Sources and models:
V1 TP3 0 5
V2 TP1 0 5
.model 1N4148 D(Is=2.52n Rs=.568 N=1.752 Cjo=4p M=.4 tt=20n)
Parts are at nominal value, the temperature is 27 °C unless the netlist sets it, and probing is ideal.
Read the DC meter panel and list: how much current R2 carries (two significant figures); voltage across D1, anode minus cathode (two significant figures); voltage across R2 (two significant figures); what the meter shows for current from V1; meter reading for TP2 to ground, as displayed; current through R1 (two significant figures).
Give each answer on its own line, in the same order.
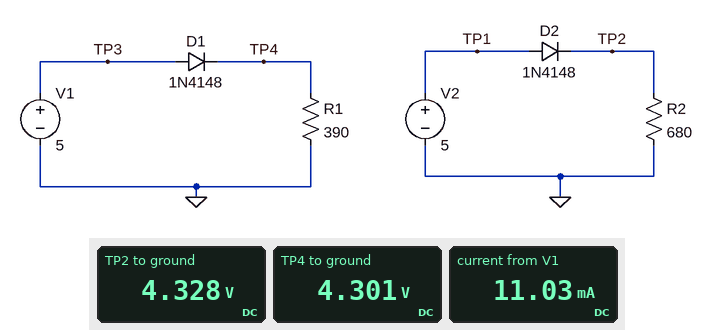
6.4 mA
700 mV
4.3 V
11.03 mA
4.328 V
11 mA
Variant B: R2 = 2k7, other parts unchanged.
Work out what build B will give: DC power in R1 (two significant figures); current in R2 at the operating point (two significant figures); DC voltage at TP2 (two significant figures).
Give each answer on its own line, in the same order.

47 mW
1.6 mA
4.4 V
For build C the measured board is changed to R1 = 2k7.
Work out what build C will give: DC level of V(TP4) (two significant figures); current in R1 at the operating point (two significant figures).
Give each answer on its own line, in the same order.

4.4 V
1.6 mA
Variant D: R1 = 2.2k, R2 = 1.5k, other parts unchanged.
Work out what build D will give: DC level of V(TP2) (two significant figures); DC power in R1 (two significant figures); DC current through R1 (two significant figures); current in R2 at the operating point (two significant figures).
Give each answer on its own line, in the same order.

4.4 V
8.7 mW
2.0 mA
2.9 mA
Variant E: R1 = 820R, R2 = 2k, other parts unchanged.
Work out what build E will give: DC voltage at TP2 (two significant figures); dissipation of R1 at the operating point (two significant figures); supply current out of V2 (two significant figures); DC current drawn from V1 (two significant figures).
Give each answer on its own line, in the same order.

4.4 V
23 mW
2.2 mA
5.3 mA
